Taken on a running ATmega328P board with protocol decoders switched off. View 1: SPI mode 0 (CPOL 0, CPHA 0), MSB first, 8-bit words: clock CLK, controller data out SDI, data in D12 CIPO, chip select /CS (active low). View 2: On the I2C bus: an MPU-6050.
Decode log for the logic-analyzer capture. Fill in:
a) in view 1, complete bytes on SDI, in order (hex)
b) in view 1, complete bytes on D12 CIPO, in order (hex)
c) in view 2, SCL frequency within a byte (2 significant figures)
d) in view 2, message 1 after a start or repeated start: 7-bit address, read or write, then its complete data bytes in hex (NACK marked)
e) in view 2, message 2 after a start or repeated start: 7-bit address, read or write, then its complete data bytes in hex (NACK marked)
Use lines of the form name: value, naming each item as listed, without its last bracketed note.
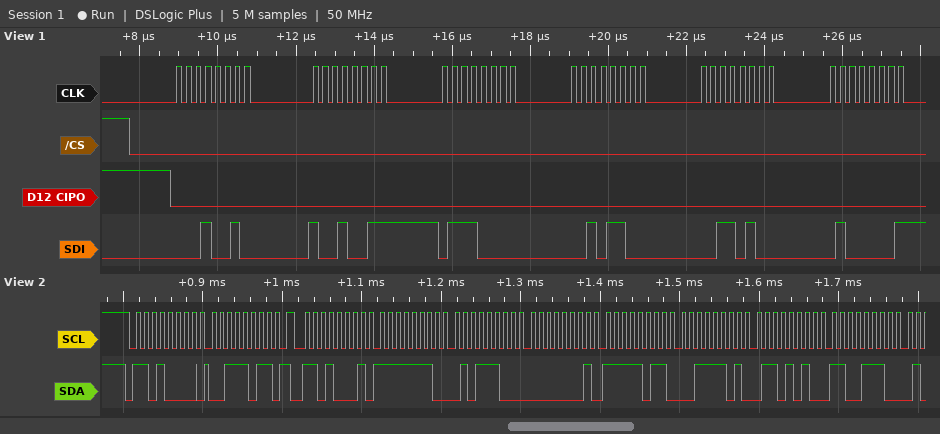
in view 1, complete bytes on SDI, in order: 0x12 0x93 0x70 0x2C 0x34 0x41
in view 1, complete bytes on D12 CIPO, in order: 0x00 0x00 0x00 0x00 0x00 0x00
in view 2, SCL frequency within a byte: 100 kHz
in view 2, message 1 after a start or repeated start: 7-bit address, read or write, then its complete data bytes in hex: 0x68 write: 3B
in view 2, message 2 after a start or repeated start: 7-bit address, read or write, then its complete data bytes in hex: 0x68 read: FE 5C 01 FB 3D 6A CE
